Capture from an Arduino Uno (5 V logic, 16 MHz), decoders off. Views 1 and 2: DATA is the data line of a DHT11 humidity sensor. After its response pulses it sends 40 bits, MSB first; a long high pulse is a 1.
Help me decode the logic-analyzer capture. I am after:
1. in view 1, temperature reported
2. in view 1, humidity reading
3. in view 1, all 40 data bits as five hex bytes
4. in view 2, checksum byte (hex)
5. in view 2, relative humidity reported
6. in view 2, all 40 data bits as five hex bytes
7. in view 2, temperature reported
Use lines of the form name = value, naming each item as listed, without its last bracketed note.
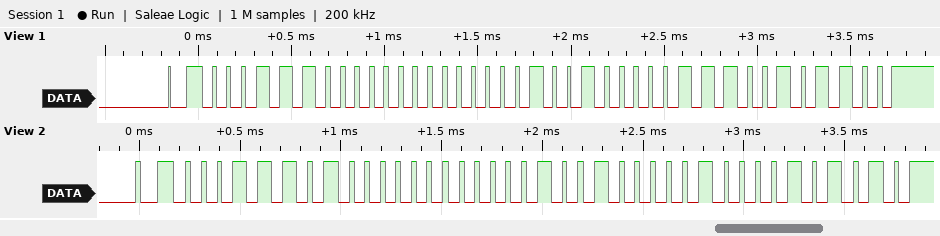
in view 1, temperature reported = 9.7 °C
in view 1, humidity reading = 28 %
in view 1, all 40 data bits as five hex bytes = 1C 00 09 07 2C
in view 2, checksum byte = 0x2A
in view 2, relative humidity reported = 29 %
in view 2, all 40 data bits as five hex bytes = 1D 00 09 04 2A
in view 2, temperature reported = 9.4 °C
